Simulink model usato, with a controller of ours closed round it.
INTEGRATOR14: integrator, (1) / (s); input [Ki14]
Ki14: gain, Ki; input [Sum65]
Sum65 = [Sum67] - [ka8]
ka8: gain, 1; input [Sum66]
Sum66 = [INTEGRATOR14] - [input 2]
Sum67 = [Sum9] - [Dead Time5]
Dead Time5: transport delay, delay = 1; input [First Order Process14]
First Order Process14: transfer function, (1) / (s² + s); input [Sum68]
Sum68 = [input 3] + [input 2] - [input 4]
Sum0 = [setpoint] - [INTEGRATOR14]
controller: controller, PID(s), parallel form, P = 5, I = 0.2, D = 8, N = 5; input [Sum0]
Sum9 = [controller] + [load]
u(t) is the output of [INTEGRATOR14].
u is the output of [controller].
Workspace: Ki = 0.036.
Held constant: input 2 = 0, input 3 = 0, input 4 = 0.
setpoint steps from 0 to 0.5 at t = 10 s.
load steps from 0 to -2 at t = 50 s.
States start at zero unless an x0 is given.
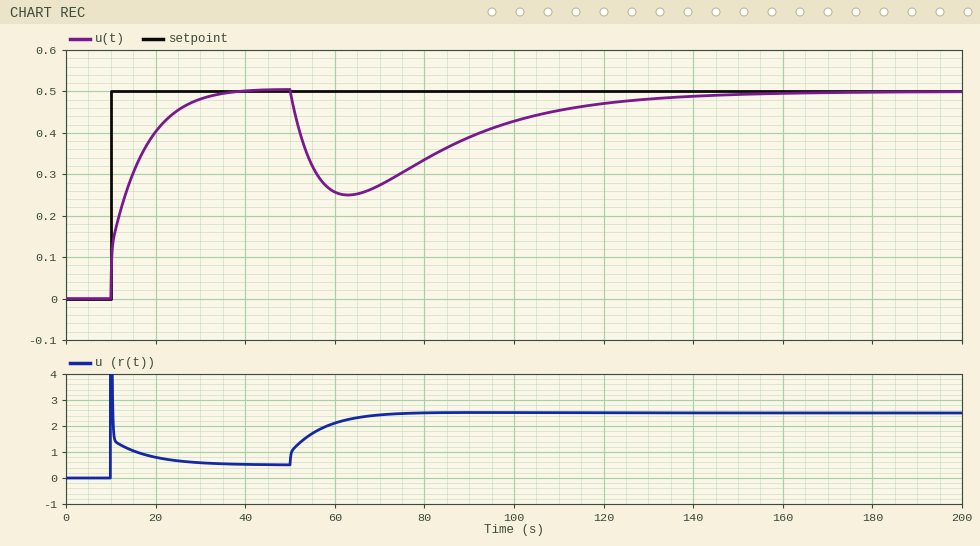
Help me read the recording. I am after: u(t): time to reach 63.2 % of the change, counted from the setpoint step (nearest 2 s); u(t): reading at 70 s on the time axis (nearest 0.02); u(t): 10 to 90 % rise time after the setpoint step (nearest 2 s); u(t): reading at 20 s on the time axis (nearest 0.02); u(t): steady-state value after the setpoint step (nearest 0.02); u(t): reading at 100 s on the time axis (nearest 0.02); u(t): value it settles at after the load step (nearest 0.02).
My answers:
6 s
0.28
14 s
0.40
0.50
0.42
0.50
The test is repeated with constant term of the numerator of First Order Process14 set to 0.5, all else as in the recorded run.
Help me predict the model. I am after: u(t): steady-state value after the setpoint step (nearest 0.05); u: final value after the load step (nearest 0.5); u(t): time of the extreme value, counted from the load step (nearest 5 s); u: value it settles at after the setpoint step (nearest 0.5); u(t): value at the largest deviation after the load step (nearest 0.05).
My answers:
0.50
2.5
15 s
0.5
0.25
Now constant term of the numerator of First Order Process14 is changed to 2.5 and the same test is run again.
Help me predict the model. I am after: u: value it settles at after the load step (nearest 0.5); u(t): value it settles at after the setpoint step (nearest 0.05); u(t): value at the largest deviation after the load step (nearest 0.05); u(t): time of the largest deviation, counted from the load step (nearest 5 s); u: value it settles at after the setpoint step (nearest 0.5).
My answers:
2.5
0.50
0.25
15 s
0.5
